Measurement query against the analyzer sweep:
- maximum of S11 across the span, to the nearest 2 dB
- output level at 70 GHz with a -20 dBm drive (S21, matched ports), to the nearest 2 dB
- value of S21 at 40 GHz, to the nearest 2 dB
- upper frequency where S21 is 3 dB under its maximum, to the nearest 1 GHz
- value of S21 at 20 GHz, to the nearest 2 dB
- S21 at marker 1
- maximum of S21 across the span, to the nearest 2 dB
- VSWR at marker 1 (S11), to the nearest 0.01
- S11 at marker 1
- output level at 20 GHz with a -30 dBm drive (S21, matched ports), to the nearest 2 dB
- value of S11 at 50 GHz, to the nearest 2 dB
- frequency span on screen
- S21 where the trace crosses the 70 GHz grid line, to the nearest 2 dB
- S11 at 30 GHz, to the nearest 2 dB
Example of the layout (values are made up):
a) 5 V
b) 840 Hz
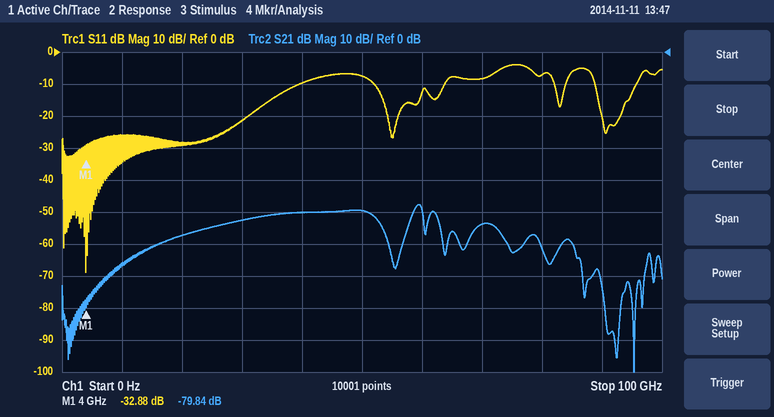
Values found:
a) -4 dB
b) -74 dBm
c) -50 dB
d) 60 GHz
e) -58 dB
f) -79.84 dB
g) -48 dB
h) 1.05
i) -32.88 dB
j) -88 dBm
k) -8 dB
l) 100 GHz
m) -54 dB
n) -22 dB
